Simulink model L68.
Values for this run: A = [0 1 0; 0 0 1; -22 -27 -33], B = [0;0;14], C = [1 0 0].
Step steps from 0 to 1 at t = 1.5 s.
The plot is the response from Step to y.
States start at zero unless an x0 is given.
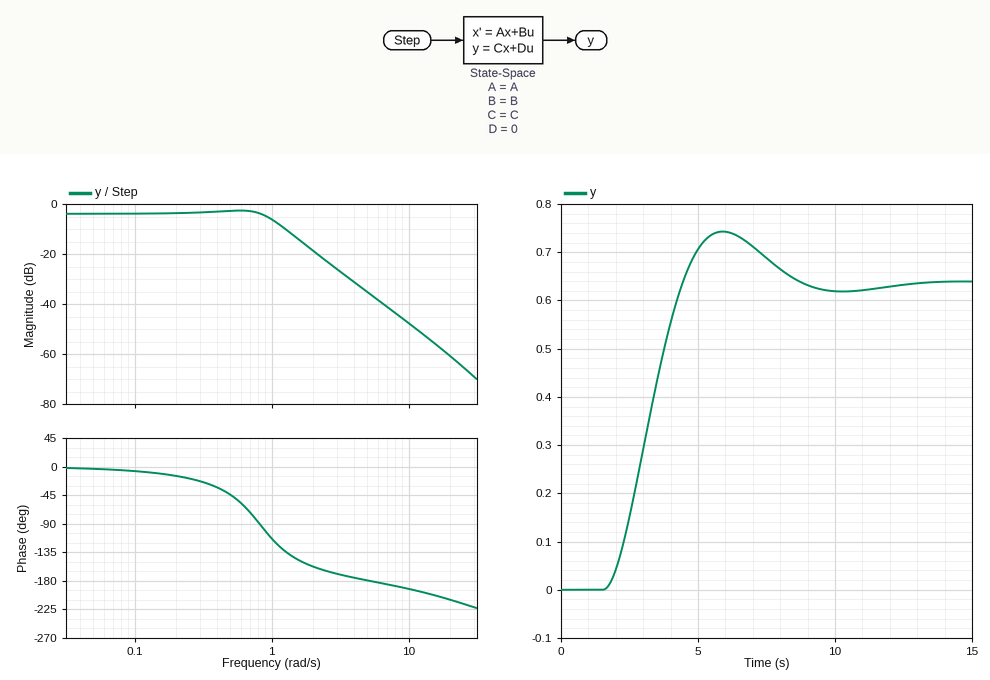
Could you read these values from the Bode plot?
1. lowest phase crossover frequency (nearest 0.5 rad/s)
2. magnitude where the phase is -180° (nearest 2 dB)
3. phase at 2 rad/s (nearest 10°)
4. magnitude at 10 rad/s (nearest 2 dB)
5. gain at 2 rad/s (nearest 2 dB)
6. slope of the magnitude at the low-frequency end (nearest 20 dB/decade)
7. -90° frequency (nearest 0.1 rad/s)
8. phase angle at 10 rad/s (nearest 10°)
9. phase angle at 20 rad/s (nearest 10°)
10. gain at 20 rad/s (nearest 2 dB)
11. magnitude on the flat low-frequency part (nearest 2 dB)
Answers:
5.0 rad/s
-36 dB
-160°
-48 dB
-18 dB
0 dB/decade
0.8 rad/s
-190°
-210°
-60 dB
-4 dB
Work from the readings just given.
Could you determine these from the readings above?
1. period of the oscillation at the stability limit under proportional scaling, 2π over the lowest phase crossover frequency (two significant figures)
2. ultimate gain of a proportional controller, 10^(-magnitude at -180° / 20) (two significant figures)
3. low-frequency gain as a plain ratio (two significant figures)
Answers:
1.3 s
63
0.63
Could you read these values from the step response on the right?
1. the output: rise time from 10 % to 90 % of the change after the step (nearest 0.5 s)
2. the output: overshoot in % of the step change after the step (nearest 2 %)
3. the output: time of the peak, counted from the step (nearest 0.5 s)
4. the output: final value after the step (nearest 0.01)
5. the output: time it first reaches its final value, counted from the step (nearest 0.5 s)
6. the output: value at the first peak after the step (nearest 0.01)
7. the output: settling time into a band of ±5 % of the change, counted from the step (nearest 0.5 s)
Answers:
2.0 s
16 %
4.5 s
0.64
3.0 s
0.74
6.5 s
